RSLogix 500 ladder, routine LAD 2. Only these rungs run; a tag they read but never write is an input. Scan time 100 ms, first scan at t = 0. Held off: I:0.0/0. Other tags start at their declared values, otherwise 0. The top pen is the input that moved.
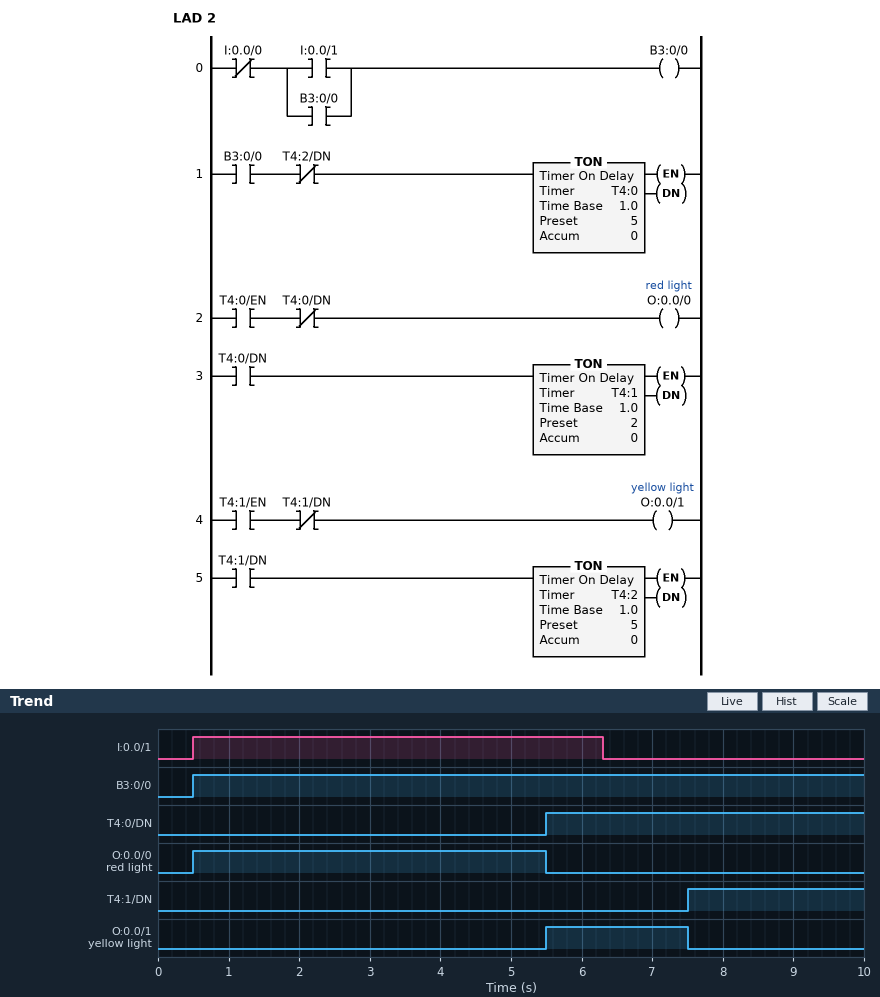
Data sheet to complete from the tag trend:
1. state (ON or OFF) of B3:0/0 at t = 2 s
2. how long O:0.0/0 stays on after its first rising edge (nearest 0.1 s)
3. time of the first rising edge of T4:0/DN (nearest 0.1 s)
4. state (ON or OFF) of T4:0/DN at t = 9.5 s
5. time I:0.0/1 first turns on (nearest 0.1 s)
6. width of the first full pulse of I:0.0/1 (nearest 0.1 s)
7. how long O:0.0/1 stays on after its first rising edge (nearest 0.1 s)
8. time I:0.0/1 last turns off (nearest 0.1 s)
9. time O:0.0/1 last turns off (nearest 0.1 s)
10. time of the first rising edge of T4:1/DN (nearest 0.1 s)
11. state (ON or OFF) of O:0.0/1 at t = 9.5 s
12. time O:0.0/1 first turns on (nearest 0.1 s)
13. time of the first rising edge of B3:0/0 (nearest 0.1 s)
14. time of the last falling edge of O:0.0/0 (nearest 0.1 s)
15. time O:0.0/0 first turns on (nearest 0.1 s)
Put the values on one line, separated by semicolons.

ON; 5.0 s; 5.5 s; ON; 0.5 s; 5.8 s; 2.0 s; 6.3 s; 7.5 s; 7.5 s; OFF; 5.5 s; 0.5 s; 5.5 s; 0.5 s
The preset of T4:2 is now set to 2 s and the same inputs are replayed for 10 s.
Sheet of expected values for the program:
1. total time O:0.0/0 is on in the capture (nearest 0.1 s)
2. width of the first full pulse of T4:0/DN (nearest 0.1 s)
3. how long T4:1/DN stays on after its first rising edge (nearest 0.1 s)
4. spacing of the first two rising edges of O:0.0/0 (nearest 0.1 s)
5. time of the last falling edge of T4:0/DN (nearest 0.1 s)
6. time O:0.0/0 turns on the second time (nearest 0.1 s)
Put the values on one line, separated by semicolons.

5.3 s; 4.1 s; 2.1 s; 9.2 s; 9.6 s; 9.7 s
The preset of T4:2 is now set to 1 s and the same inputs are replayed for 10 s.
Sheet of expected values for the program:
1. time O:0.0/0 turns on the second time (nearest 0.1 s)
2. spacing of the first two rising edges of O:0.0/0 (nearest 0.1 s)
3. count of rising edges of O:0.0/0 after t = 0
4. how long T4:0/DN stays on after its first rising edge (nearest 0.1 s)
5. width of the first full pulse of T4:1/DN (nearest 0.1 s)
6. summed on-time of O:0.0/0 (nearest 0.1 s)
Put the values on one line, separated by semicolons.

8.7 s; 8.2 s; 2; 3.1 s; 1.1 s; 6.3 s
